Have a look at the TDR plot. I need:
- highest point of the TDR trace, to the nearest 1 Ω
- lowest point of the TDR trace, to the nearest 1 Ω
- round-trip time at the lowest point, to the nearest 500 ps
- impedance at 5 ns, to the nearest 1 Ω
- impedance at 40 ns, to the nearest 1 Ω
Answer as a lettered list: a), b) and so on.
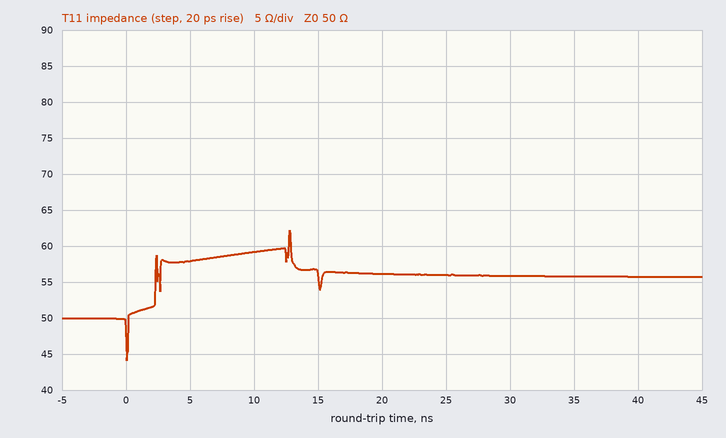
a) 62 Ω
b) 44 Ω
c) 0.0 ns
d) 58 Ω
e) 56 Ω
